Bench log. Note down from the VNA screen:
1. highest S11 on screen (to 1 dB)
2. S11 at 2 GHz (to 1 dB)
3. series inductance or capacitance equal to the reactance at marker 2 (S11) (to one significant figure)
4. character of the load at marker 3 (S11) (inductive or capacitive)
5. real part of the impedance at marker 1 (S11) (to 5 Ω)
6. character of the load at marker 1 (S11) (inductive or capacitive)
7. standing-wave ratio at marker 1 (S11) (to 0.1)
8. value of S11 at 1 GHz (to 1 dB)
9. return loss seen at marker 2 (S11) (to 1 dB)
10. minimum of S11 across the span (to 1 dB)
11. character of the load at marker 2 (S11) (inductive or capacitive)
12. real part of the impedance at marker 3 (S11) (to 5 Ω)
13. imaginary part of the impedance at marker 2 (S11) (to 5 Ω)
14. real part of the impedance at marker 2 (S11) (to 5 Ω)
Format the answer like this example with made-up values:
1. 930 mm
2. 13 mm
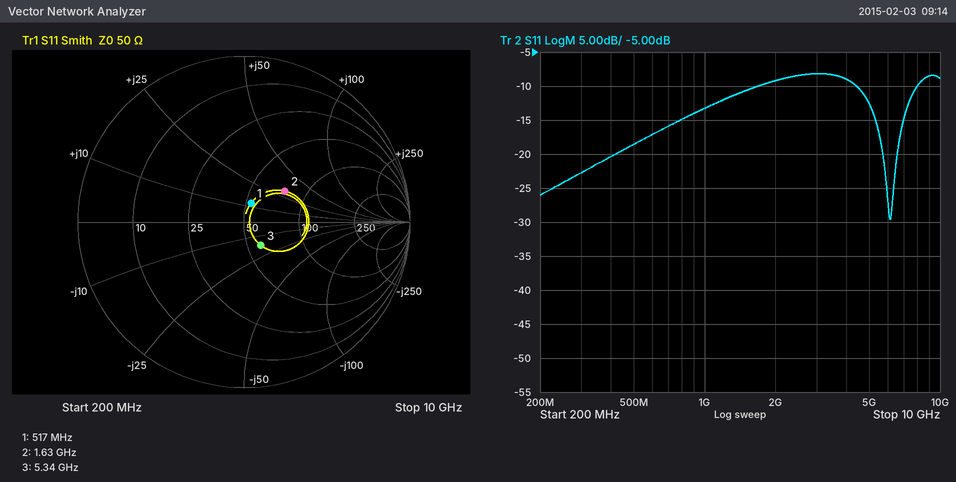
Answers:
1. -8 dB
2. -9 dB
3. 3 nH
4. capacitive
5. 55 Ω
6. inductive
7. 1.3
8. -13 dB
9. 10 dB
10. -30 dB
11. inductive
12. 60 Ω
13. +30 Ω
14. 75 Ω
